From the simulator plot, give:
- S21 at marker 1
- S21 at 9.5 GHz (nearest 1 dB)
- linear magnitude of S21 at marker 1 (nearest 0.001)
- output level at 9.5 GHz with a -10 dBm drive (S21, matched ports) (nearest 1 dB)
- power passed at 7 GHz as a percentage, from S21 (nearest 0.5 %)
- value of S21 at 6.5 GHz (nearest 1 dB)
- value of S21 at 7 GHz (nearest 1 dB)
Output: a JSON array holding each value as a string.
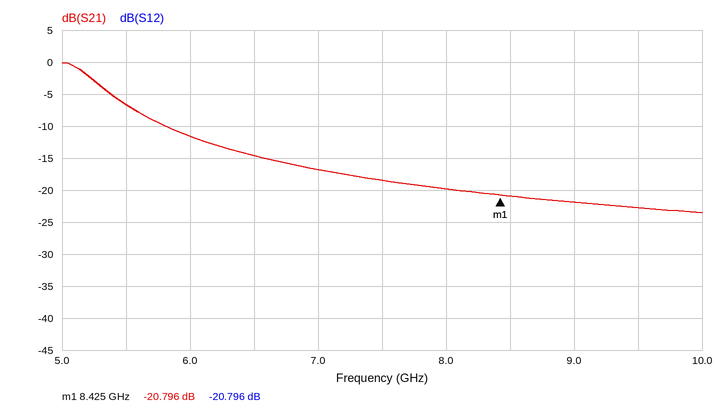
["-20.796 dB", "-23 dB", "0.091", "-33 dBm", "2.0 %", "-15 dB", "-17 dB"]
